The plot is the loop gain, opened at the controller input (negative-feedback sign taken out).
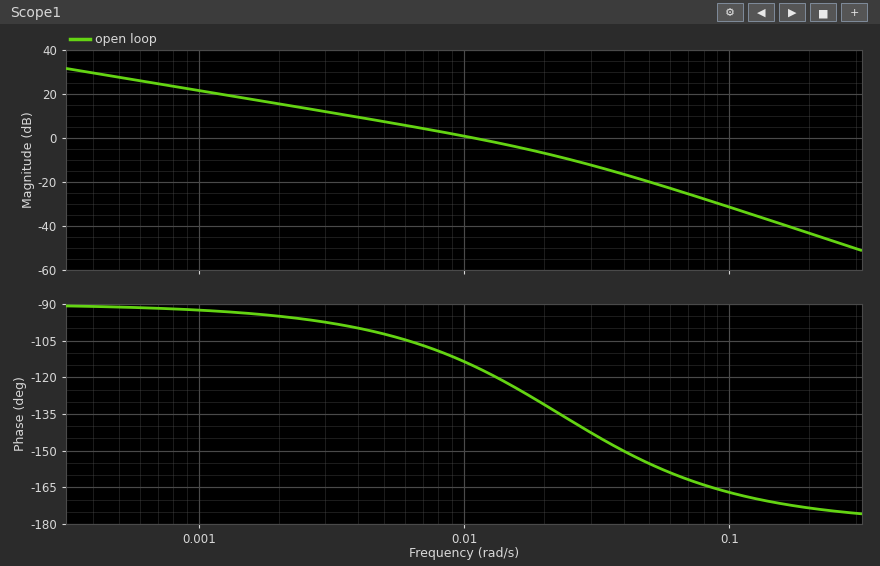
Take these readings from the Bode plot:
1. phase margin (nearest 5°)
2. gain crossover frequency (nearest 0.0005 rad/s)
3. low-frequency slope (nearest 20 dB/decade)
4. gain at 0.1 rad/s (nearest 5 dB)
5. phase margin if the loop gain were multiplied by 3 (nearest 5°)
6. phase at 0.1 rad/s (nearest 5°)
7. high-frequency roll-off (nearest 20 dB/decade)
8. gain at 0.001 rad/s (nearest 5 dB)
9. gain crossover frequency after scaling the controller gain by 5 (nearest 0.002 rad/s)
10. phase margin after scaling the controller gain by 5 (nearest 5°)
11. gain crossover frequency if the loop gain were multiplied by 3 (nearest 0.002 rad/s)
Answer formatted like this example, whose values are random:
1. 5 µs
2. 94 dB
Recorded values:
1. 65°
2. 0.0110 rad/s
3. -20 dB/decade
4. -30 dB
5. 45°
6. -165°
7. -40 dB/decade
8. 20 dB
9. 0.034 rad/s
10. 35°
11. 0.024 rad/s
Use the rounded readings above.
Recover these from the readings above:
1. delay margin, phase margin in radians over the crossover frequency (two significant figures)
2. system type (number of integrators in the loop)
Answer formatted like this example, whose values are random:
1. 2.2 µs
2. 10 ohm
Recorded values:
1. 100 s
2. 1
